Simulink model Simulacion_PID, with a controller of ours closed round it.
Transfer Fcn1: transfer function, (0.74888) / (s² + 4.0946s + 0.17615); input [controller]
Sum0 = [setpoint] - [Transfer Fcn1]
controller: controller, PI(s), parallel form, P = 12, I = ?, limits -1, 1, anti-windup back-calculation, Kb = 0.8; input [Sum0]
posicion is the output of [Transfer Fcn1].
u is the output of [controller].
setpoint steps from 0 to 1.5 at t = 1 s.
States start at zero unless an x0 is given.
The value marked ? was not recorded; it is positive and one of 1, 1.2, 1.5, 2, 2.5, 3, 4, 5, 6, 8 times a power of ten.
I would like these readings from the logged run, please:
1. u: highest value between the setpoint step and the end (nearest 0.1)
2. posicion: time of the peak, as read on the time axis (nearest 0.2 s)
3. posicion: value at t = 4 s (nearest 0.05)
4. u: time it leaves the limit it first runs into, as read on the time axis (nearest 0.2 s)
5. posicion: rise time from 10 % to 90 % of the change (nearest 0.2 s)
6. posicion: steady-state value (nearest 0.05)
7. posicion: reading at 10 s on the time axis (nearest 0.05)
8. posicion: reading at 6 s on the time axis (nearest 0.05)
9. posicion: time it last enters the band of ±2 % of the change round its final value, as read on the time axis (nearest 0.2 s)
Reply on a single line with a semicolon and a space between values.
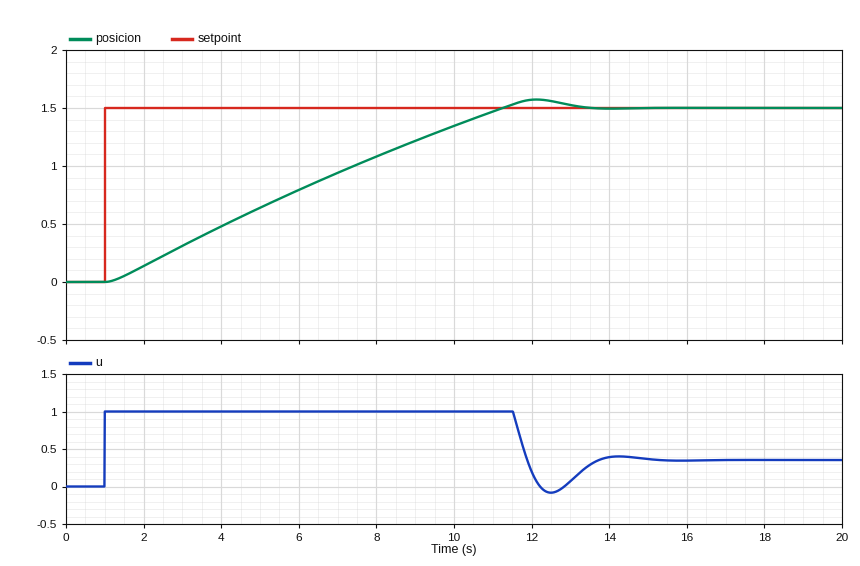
1.0; 12.2 s; 0.50; 11.6 s; 8.0 s; 1.50; 1.35; 0.80; 13.0 s
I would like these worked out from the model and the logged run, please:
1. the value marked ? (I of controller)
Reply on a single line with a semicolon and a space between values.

12
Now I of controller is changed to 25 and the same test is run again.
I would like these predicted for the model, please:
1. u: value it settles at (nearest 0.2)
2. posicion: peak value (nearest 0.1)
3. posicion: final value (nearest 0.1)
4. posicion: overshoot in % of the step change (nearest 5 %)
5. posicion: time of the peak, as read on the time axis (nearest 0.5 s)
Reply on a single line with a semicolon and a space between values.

0.4; 1.6; 1.5; 10 %; 12.5 s
